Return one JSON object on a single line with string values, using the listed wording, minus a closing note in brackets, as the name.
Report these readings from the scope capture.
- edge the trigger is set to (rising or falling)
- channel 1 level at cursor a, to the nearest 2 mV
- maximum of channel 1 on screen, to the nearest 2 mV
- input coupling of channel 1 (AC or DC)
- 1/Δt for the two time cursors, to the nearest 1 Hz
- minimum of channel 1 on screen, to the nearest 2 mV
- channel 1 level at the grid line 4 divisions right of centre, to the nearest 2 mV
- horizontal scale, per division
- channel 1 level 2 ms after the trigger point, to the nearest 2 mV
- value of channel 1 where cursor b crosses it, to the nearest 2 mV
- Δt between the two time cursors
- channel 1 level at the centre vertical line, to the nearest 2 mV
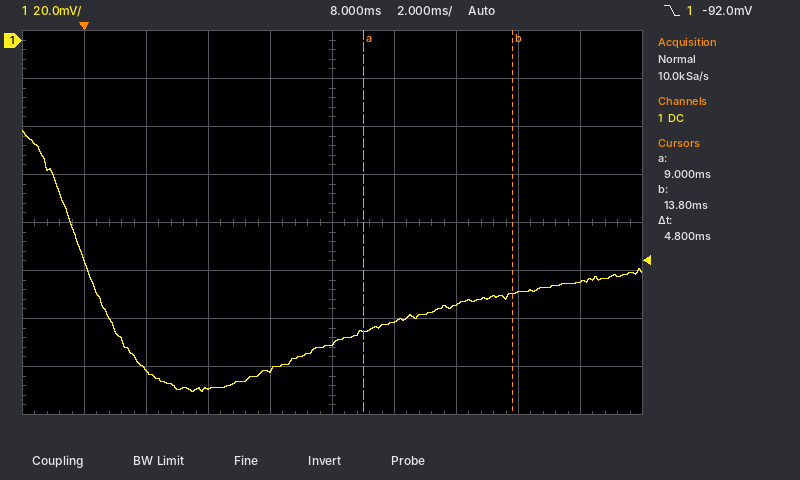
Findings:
{"edge the trigger is set to": "falling", "channel 1 level at cursor a, to the nearest 2 mV": "-122 mV", "maximum of channel 1 on screen, to the nearest 2 mV": "-38 mV", "input coupling of channel 1": "DC", "1/Δt for the two time cursors, to the nearest 1 Hz": "208 Hz", "minimum of channel 1 on screen, to the nearest 2 mV": "-146 mV", "channel 1 level at the grid line 4 divisions right of centre, to the nearest 2 mV": "-100 mV", "horizontal scale, per division": "2 ms", "channel 1 level 2 ms after the trigger point, to the nearest 2 mV": "-138 mV", "value of channel 1 where cursor b crosses it, to the nearest 2 mV": "-106 mV", "Δt between the two time cursors": "4.8 ms", "channel 1 level at the centre vertical line, to the nearest 2 mV": "-126 mV"}
